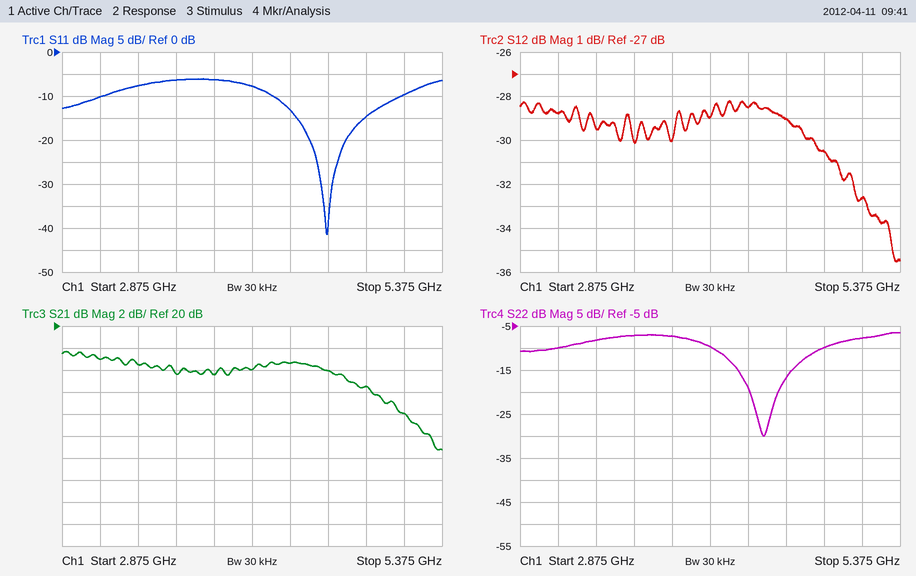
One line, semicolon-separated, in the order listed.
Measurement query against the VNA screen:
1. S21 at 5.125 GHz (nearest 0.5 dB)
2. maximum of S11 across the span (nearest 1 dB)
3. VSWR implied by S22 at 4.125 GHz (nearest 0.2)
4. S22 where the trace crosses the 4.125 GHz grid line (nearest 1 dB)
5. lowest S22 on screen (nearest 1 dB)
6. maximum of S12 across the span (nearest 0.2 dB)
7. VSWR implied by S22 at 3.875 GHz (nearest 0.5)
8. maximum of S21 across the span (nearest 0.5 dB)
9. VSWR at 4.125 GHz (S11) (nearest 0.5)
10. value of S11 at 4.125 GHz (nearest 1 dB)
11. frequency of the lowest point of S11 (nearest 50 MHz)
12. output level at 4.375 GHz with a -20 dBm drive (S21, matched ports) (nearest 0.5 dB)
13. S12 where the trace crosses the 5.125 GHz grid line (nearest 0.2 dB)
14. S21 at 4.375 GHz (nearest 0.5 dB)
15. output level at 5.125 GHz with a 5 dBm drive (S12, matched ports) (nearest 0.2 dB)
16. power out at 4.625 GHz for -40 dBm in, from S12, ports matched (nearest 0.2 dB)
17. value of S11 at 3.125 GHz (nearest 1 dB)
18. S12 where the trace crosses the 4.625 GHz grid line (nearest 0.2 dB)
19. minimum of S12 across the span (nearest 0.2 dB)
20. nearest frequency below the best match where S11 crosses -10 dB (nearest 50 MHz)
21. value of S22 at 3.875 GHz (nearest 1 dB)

12.0 dB; -6 dB; 2.0; -10 dB; -30 dB; -28.2 dB; 2.5; 17.5 dB; 2.5; -8 dB; 4.60 GHz; -3.5 dBm; -32.6 dB; 16.5 dB; -27.6 dBm; -69.0 dBm; -10 dB; -29.0 dB; -35.6 dB; 4.25 GHz; -7 dB
